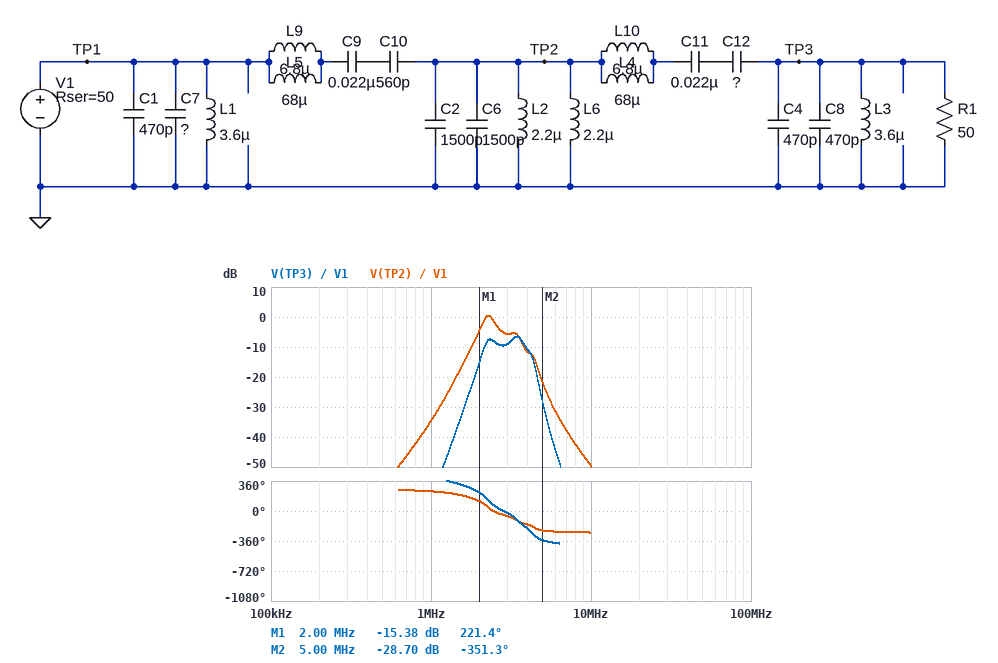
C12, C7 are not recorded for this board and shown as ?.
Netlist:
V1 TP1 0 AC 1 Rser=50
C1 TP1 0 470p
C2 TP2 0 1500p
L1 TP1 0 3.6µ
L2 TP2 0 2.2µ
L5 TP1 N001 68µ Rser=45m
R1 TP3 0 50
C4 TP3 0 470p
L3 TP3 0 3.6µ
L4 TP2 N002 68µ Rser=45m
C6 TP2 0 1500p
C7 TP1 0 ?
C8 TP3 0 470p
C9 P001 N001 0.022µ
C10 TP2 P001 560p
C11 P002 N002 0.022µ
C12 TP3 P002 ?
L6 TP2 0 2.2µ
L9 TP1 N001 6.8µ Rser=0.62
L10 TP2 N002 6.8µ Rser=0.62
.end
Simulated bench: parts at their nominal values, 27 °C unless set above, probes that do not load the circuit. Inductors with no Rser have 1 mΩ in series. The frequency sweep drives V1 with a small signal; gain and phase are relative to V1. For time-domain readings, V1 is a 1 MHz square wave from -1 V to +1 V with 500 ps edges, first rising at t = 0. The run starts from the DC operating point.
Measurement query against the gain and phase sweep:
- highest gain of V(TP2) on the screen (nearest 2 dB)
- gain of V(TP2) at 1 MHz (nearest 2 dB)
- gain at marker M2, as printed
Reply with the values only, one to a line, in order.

0 dB
-34 dB
-28.70 dB
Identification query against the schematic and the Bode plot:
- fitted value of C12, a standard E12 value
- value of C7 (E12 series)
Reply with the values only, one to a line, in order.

330 pF
1.2 nF
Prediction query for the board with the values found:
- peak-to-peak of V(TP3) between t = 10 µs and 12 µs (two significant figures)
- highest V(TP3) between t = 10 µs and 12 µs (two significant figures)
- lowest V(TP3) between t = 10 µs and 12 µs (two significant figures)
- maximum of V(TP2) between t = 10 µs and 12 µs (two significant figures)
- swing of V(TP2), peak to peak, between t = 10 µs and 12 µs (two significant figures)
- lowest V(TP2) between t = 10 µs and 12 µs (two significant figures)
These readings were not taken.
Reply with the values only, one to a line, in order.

320 mV
160 mV
-160 mV
240 mV
490 mV
-240 mV
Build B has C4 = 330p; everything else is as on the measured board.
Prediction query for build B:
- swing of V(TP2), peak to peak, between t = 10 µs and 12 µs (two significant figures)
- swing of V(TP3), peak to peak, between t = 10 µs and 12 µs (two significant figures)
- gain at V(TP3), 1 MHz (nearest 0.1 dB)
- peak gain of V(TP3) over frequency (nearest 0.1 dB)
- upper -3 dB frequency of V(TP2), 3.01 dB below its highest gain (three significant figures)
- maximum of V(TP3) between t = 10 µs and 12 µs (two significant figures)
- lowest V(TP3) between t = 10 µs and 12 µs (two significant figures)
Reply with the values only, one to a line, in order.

480 mV
330 mV
-60.2 dB
-6.3 dB
2.53 MHz
170 mV
-170 mV
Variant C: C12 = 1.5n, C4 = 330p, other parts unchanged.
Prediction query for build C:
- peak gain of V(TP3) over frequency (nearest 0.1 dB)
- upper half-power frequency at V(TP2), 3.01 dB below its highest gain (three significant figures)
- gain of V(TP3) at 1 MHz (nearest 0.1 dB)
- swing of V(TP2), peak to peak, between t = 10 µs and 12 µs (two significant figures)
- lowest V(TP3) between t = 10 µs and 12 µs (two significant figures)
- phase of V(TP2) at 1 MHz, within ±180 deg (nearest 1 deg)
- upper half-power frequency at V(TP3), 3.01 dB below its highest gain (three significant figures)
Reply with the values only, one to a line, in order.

-6.9 dB
3.90 MHz
-41.2 dB
610 mV
-160 mV
-126 deg
3.87 MHz
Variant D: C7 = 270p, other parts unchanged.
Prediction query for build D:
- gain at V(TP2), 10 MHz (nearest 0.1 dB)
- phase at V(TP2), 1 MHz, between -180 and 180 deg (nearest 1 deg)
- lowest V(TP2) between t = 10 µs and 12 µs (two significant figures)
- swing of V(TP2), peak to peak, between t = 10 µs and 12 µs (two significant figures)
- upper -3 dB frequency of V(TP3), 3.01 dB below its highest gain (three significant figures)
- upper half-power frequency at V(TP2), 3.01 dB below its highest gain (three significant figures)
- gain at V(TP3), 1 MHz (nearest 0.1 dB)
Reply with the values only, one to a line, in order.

-42.5 dB
-120 deg
-300 mV
600 mV
4.25 MHz
3.01 MHz
-61.2 dB
